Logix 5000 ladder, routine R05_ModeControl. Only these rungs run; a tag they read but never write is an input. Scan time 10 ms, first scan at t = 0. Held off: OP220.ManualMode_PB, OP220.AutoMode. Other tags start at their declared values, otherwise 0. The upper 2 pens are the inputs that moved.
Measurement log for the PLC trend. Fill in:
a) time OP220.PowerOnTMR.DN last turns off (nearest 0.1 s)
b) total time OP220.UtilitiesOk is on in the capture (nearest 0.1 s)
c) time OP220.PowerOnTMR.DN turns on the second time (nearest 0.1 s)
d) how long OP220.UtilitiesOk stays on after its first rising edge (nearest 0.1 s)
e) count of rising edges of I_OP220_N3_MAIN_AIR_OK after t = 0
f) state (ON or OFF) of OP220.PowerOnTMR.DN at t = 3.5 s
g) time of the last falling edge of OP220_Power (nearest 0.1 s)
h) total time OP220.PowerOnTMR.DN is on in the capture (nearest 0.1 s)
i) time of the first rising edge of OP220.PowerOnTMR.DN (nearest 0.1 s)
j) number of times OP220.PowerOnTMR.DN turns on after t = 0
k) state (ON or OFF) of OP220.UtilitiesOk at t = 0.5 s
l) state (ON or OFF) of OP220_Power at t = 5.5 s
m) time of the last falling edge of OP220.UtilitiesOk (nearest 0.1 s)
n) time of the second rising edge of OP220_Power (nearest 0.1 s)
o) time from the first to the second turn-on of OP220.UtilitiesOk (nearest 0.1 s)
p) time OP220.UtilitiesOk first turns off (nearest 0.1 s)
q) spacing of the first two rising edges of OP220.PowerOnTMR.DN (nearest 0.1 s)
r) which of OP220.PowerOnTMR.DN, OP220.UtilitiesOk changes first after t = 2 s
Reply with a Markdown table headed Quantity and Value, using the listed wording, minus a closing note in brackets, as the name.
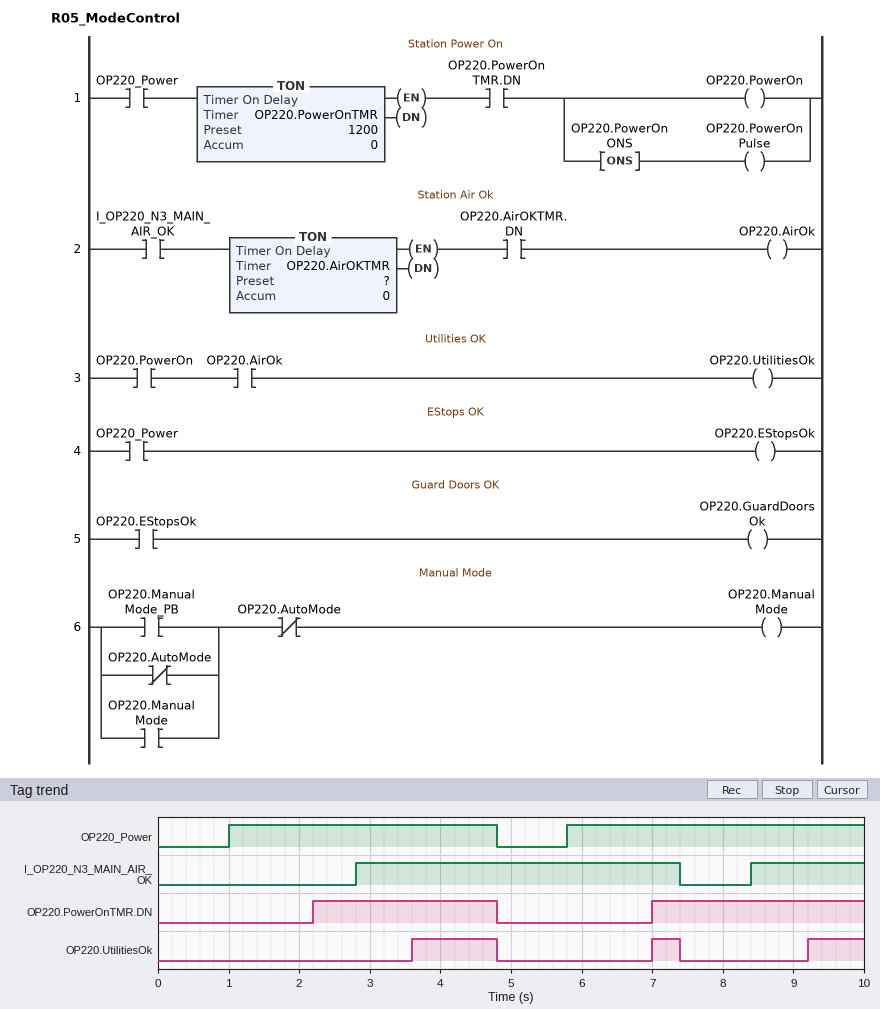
| Quantity | Value |
|---|---|
| time OP220.PowerOnTMR.DN last turns off | 4.8 s |
| total time OP220.UtilitiesOk is on in the capture | 2.4 s |
| time OP220.PowerOnTMR.DN turns on the second time | 7.0 s |
| how long OP220.UtilitiesOk stays on after its first rising edge | 1.2 s |
| count of rising edges of I_OP220_N3_MAIN_AIR_OK after t = 0 | 2 |
| state (ON or OFF) of OP220.PowerOnTMR.DN at t = 3.5 s | ON |
| time of the last falling edge of OP220_Power | 4.8 s |
| total time OP220.PowerOnTMR.DN is on in the capture | 5.6 s |
| time of the first rising edge of OP220.PowerOnTMR.DN | 2.2 s |
| number of times OP220.PowerOnTMR.DN turns on after t = 0 | 2 |
| state (ON or OFF) of OP220.UtilitiesOk at t = 0.5 s | OFF |
| state (ON or OFF) of OP220_Power at t = 5.5 s | OFF |
| time of the last falling edge of OP220.UtilitiesOk | 7.4 s |
| time of the second rising edge of OP220_Power | 5.8 s |
| time from the first to the second turn-on of OP220.UtilitiesOk | 3.4 s |
| time OP220.UtilitiesOk first turns off | 4.8 s |
| spacing of the first two rising edges of OP220.PowerOnTMR.DN | 4.8 s |
| which of OP220.PowerOnTMR.DN, OP220.UtilitiesOk changes first after t = 2 s | OP220.PowerOnTMR.DN |
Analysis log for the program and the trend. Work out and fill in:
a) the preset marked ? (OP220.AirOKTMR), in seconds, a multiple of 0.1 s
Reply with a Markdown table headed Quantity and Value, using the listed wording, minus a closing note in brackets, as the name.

| Quantity | Value |
|---|---|
| the preset marked ? (OP220.AirOKTMR), in seconds, a multiple of 0.1 s | 0.8 s |
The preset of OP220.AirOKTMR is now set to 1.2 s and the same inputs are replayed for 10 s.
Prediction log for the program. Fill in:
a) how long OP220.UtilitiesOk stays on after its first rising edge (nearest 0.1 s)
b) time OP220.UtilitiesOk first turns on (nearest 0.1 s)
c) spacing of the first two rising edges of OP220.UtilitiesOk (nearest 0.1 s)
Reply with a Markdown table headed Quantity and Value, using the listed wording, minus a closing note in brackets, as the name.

| Quantity | Value |
|---|---|
| how long OP220.UtilitiesOk stays on after its first rising edge | 0.8 s |
| time OP220.UtilitiesOk first turns on | 4.0 s |
| spacing of the first two rising edges of OP220.UtilitiesOk | 3.0 s |
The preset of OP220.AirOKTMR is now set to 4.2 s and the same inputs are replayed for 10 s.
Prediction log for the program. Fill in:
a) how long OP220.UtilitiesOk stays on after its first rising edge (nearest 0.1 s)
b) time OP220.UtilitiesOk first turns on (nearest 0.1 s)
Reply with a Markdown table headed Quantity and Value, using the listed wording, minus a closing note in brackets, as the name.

| Quantity | Value |
|---|---|
| how long OP220.UtilitiesOk stays on after its first rising edge | 0.4 s |
| time OP220.UtilitiesOk first turns on | 7.0 s |
